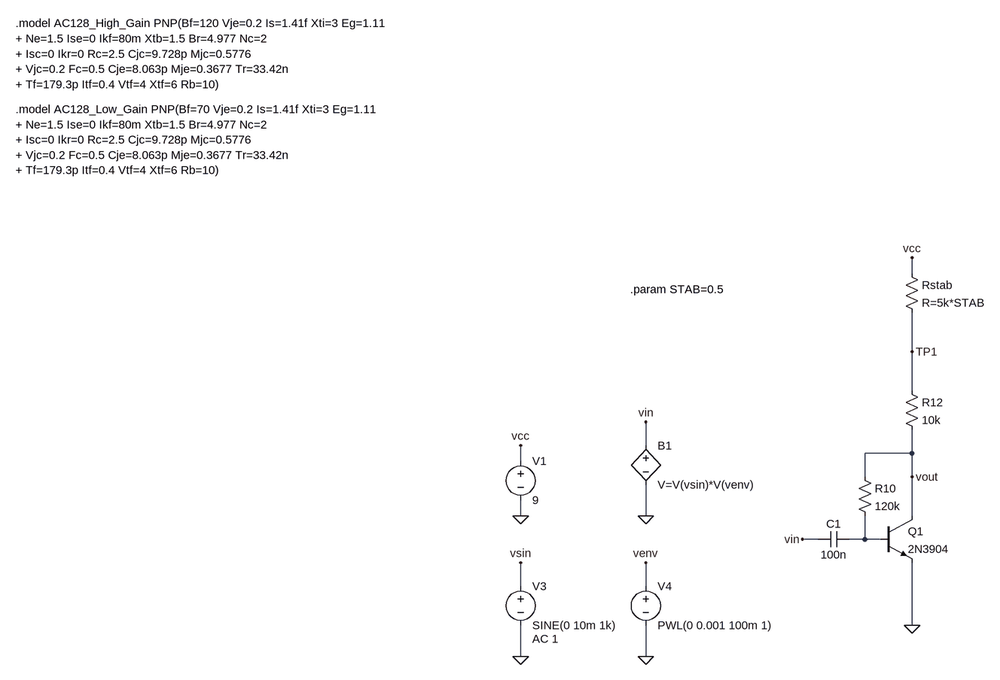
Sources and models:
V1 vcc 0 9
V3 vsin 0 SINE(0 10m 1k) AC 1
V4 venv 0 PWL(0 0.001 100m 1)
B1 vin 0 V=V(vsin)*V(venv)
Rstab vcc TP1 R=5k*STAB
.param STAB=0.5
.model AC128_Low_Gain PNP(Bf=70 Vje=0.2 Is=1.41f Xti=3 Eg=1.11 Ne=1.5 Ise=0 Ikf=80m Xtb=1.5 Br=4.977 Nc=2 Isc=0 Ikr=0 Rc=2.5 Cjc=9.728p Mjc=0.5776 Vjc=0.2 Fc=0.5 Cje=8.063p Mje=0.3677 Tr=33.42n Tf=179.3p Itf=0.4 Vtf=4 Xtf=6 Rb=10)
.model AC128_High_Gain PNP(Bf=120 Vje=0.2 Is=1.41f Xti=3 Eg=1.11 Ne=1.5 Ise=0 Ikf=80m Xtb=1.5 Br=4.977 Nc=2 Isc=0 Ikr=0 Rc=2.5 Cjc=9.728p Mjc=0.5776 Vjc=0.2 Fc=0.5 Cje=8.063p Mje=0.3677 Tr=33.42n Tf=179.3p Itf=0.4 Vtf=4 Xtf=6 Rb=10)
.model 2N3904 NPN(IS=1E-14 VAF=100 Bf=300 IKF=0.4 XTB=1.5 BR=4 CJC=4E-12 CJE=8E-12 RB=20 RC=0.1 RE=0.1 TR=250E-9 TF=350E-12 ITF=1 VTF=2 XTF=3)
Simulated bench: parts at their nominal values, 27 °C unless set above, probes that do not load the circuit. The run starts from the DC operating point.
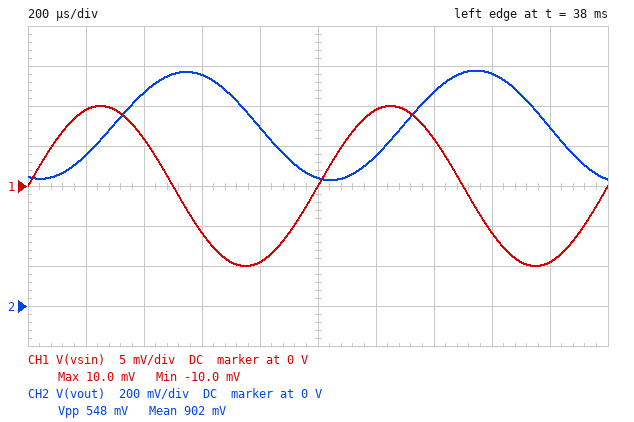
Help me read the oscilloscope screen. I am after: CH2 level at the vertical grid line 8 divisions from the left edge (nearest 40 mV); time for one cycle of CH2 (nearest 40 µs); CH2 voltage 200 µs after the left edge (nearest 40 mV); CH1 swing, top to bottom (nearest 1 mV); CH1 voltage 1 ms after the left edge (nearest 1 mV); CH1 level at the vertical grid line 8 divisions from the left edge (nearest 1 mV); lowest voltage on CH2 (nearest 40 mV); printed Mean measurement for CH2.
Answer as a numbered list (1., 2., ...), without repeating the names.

1. 1.16 V
2. 1.00 ms
3. 760 mV
4. 20 mV
5. 0 V
6. -6 mV
7. 640 mV
8. 902 mV
